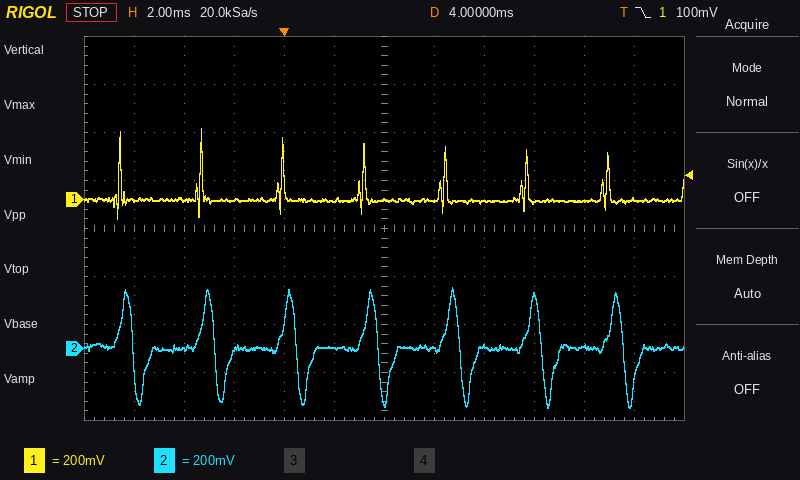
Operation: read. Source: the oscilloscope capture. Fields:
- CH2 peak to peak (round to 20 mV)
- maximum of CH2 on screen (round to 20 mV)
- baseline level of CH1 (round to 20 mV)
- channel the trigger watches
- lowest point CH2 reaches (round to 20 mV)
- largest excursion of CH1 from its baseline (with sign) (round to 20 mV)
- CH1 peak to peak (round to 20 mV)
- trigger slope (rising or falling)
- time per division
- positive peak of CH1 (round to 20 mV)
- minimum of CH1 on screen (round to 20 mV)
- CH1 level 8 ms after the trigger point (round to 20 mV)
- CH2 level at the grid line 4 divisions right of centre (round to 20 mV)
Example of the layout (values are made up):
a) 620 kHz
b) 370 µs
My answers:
a) 500 mV
b) 260 mV
c) 0 mV
d) CH1
e) -240 mV
f) +300 mV
g) 380 mV
h) falling
i) 2 ms
j) 300 mV
k) -80 mV
l) 0 mV
m) 0 mV
